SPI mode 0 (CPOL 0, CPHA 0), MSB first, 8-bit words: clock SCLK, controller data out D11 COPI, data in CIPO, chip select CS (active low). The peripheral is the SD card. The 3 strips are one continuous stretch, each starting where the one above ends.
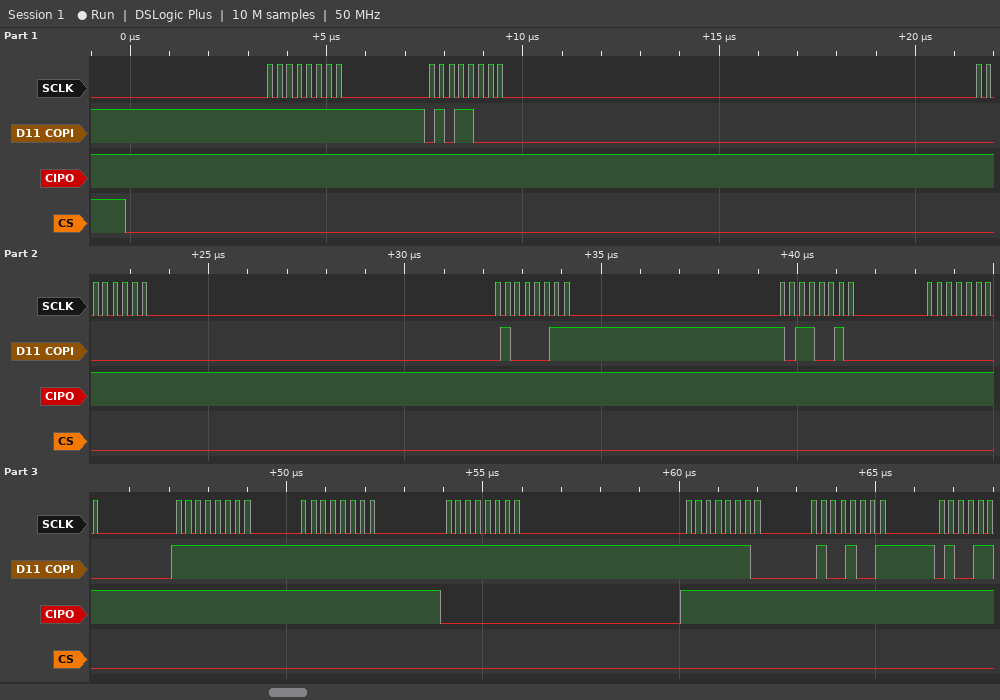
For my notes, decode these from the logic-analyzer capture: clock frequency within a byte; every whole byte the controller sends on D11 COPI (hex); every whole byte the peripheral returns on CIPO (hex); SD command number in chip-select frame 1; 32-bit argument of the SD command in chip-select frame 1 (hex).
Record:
4 MHz
FF 58 00 43 B2 00 FF FF FF FE 49
FF FF FF FF FF FF FF FF 00 FF FF
CMD24
0x0043B200
